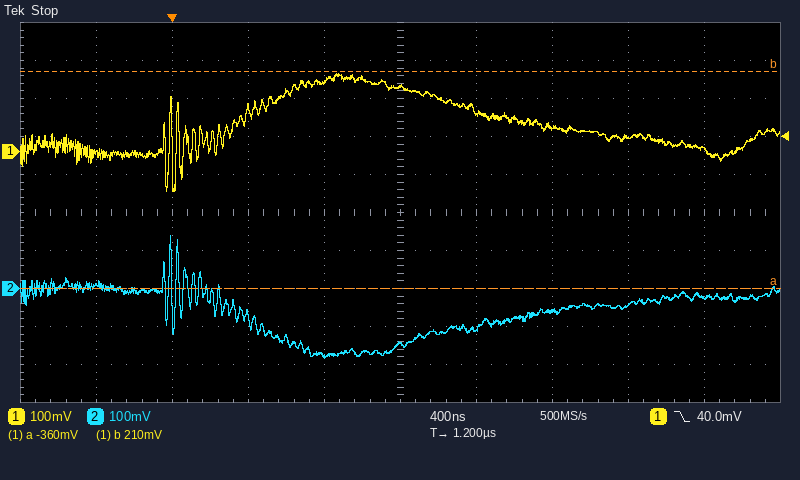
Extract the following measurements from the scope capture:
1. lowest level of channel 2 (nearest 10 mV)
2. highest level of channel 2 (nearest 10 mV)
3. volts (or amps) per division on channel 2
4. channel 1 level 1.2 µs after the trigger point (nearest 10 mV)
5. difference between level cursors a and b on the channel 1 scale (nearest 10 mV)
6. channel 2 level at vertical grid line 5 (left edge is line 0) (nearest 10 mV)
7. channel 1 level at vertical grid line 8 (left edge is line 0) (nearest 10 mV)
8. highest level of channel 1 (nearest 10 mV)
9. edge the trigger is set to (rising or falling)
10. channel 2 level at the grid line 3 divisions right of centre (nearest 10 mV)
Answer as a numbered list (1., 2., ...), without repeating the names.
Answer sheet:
1. -180 mV
2. 140 mV
3. 100 mV
4. 170 mV
5. 570 mV
6. -150 mV
7. 40 mV
8. 210 mV
9. falling
10. -40 mV
